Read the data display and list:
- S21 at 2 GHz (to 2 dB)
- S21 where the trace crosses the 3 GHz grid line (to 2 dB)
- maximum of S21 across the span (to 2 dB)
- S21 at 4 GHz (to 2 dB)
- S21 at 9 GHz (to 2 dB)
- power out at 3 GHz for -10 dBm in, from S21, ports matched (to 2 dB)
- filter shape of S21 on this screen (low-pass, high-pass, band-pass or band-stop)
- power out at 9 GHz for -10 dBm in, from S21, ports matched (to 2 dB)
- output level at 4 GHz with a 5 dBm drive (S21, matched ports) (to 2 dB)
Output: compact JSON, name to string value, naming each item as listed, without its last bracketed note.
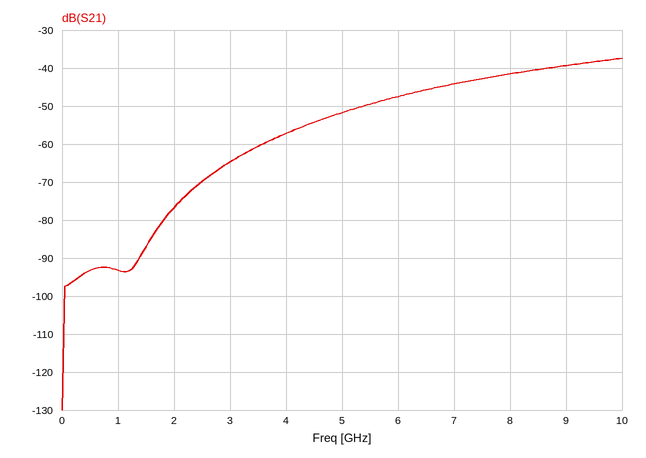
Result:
{"S21 at 2 GHz": "-76 dB", "S21 where the trace crosses the 3 GHz grid line": "-64 dB", "maximum of S21 across the span": "-38 dB", "S21 at 4 GHz": "-58 dB", "S21 at 9 GHz": "-40 dB", "power out at 3 GHz for -10 dBm in, from S21, ports matched": "-74 dBm", "filter shape of S21 on this screen": "high-pass", "power out at 9 GHz for -10 dBm in, from S21, ports matched": "-50 dBm", "output level at 4 GHz with a 5 dBm drive (S21, matched ports)": "-52 dBm"}
